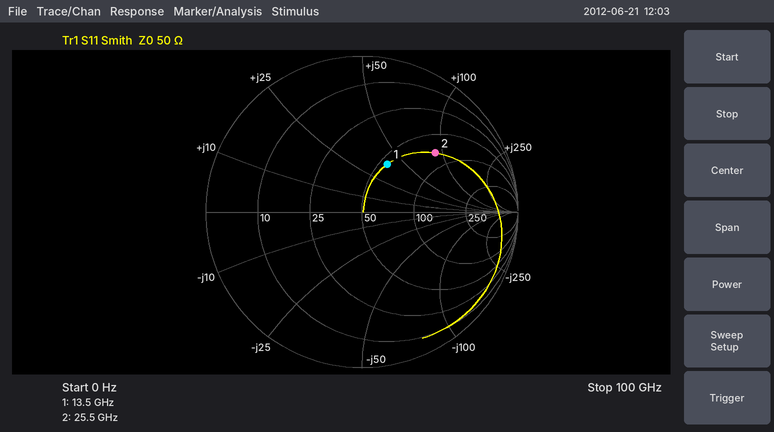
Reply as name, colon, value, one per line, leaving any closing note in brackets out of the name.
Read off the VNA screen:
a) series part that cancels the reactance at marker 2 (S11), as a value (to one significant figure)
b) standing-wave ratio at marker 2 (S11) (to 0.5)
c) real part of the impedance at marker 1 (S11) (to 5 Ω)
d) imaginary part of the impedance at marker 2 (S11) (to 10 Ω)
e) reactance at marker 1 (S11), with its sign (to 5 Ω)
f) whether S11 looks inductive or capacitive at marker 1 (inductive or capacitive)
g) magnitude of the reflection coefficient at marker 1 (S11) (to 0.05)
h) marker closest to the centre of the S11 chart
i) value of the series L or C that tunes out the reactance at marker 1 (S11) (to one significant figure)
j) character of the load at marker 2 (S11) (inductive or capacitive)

series part that cancels the reactance at marker 2 (S11), as a value: 70 fF
standing-wave ratio at marker 2 (S11): 4.0
real part of the impedance at marker 1 (S11): 55 Ω
imaginary part of the impedance at marker 2 (S11): +90 Ω
reactance at marker 1 (S11), with its sign: +40 Ω
whether S11 looks inductive or capacitive at marker 1: inductive
magnitude of the reflection coefficient at marker 1 (S11): 0.35
marker closest to the centre of the S11 chart: marker 1
value of the series L or C that tunes out the reactance at marker 1 (S11): 300 fF
character of the load at marker 2 (S11): inductive
